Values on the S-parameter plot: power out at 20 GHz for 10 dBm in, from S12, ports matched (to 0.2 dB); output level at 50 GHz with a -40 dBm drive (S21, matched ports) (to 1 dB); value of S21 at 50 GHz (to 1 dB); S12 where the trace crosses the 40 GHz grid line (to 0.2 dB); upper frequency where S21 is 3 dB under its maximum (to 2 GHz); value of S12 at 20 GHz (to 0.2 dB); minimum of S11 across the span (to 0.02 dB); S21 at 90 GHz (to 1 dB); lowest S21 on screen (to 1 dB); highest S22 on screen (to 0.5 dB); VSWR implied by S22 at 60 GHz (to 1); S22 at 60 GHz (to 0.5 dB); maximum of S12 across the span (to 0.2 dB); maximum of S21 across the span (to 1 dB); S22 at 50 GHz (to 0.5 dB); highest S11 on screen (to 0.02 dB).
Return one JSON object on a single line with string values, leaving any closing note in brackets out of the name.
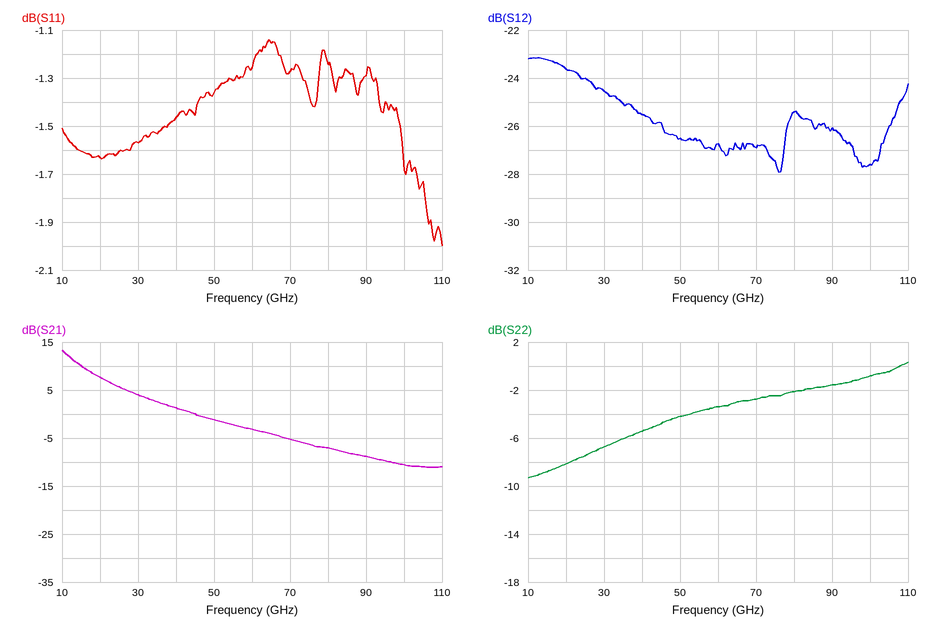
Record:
{"power out at 20 GHz for 10 dBm in, from S12, ports matched": "-13.6 dBm", "output level at 50 GHz with a -40 dBm drive (S21, matched ports)": "-41 dBm", "value of S21 at 50 GHz": "-1 dB", "S12 where the trace crosses the 40 GHz grid line": "-25.6 dB", "upper frequency where S21 is 3 dB under its maximum": "14 GHz", "value of S12 at 20 GHz": "-23.6 dB", "minimum of S11 across the span": "-2.00 dB", "S21 at 90 GHz": "-9 dB", "lowest S21 on screen": "-11 dB", "highest S22 on screen": "0.5 dB", "VSWR implied by S22 at 60 GHz": "5", "S22 at 60 GHz": "-3.5 dB", "maximum of S12 across the span": "-23.2 dB", "maximum of S21 across the span": "13 dB", "S22 at 50 GHz": "-4.0 dB", "highest S11 on screen": "-1.14 dB"}
